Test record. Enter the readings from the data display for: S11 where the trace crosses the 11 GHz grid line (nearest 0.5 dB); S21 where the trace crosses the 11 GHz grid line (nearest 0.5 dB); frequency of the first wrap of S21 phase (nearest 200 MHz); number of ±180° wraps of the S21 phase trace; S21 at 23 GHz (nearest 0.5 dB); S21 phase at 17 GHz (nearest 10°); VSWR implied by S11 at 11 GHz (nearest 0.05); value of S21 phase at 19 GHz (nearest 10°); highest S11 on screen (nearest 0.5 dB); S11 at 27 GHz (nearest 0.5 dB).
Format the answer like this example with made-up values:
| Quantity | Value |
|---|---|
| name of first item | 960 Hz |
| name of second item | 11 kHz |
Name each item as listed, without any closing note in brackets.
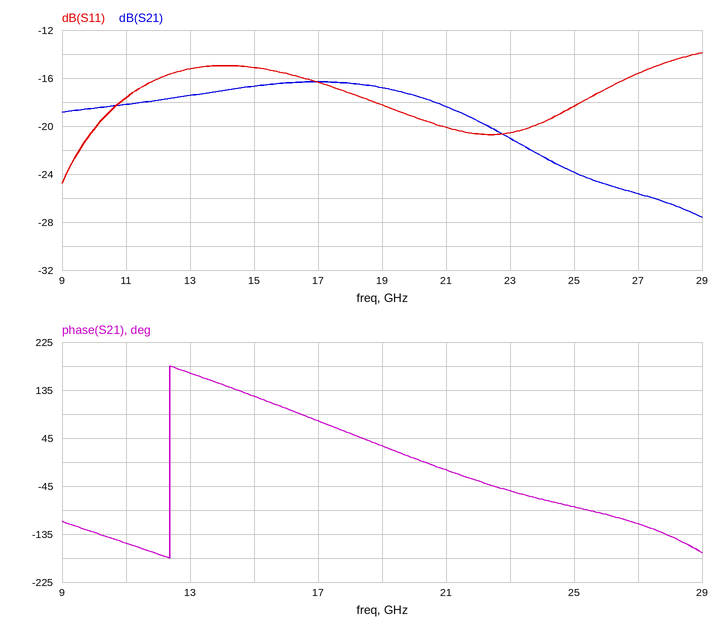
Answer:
| Quantity | Value |
|---|---|
| S11 where the trace crosses the 11 GHz grid line | -17.5 dB |
| S21 where the trace crosses the 11 GHz grid line | -18.0 dB |
| frequency of the first wrap of S21 phase | 12.4 GHz |
| number of ±180° wraps of the S21 phase trace | 1 |
| S21 at 23 GHz | -21.0 dB |
| S21 phase at 17 GHz | 80° |
| VSWR implied by S11 at 11 GHz | 1.30 |
| value of S21 phase at 19 GHz | 30° |
| highest S11 on screen | -14.0 dB |
| S11 at 27 GHz | -15.5 dB |
